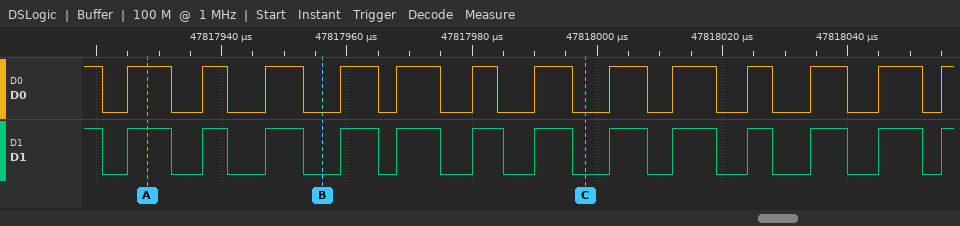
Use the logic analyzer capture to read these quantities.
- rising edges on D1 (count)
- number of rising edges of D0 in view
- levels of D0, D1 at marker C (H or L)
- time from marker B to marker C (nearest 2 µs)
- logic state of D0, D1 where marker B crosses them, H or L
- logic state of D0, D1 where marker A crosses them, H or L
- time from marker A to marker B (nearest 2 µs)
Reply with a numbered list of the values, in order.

1. 13
2. 13
3. D0=L, D1=L
4. 42 µs
5. D0=L, D1=L
6. D0=H, D1=H
7. 28 µs
